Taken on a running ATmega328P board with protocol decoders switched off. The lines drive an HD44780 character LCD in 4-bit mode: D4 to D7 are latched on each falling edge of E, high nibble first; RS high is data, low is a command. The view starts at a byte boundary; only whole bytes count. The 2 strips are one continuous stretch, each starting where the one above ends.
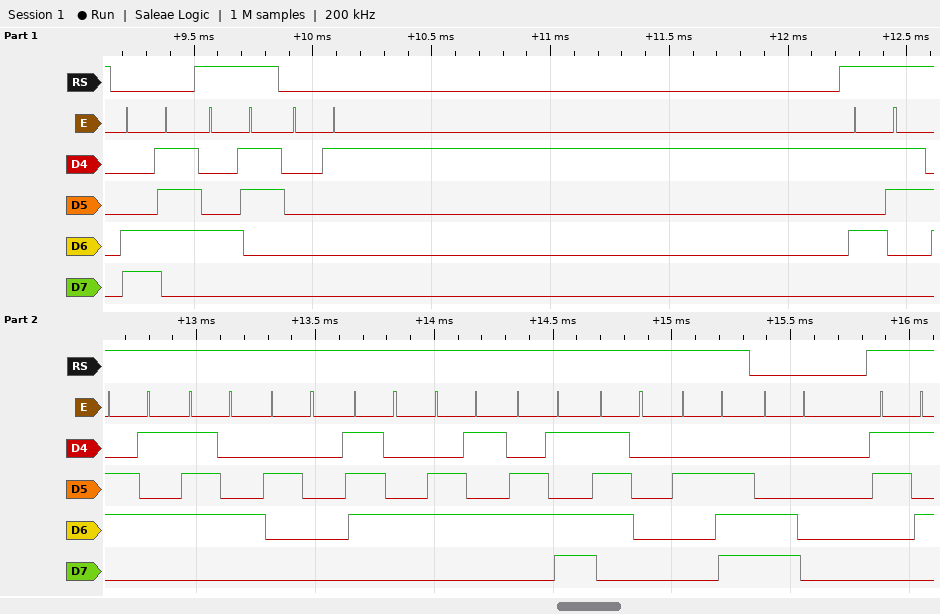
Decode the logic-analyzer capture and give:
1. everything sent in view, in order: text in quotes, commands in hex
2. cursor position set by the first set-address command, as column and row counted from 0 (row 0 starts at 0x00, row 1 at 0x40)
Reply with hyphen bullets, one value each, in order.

- 0xC7 "C" 0x01 "Set temp." 0xC0 "5"
- column 7, row 1
